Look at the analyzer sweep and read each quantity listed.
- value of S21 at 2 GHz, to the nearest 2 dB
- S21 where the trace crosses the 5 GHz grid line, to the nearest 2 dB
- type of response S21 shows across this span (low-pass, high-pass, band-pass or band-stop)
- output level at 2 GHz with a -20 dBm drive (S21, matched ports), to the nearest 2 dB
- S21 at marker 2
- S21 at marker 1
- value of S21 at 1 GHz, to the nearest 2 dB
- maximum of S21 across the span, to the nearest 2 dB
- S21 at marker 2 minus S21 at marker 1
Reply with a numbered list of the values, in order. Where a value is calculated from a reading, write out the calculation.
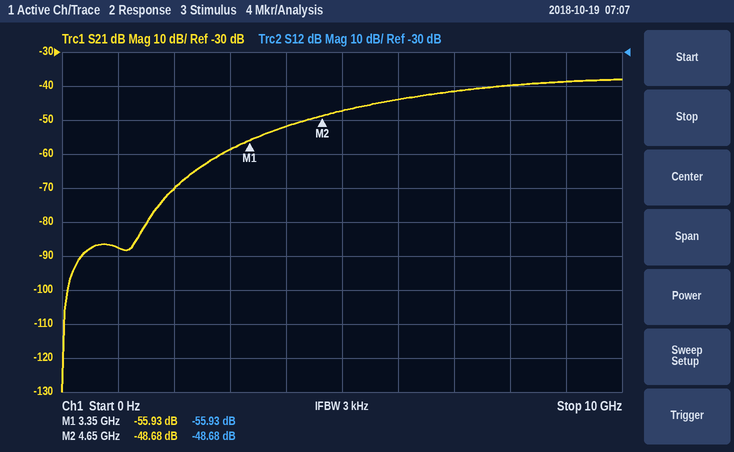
1. -70 dB
2. -48 dB
3. high-pass
4. -20 dBm + (-70 dB) = -90 dBm
5. -48.68 dB
6. -55.93 dB
7. -88 dB
8. -38 dB
9. -48.68 − (-55.93) = 7.25 dB
